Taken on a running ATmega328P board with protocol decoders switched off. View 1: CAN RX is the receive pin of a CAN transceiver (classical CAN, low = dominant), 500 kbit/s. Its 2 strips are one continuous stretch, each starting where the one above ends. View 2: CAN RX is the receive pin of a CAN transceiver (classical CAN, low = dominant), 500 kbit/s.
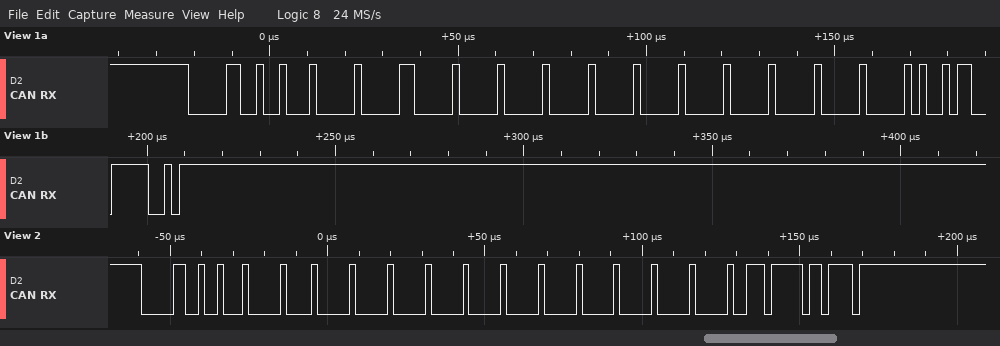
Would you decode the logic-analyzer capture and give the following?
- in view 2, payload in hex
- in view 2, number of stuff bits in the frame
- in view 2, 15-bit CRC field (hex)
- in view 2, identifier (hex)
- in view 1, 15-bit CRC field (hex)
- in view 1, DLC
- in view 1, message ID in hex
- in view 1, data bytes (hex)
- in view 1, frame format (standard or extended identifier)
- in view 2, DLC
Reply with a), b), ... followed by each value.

a) 02 00 00 00 00 00 00 00
b) 14
c) 0x77F7
d) 0x049
e) 0x4B3E
f) 8
g) 0x049
h) 01 00 00 00 00 00 00 00
i) standard
j) 8
